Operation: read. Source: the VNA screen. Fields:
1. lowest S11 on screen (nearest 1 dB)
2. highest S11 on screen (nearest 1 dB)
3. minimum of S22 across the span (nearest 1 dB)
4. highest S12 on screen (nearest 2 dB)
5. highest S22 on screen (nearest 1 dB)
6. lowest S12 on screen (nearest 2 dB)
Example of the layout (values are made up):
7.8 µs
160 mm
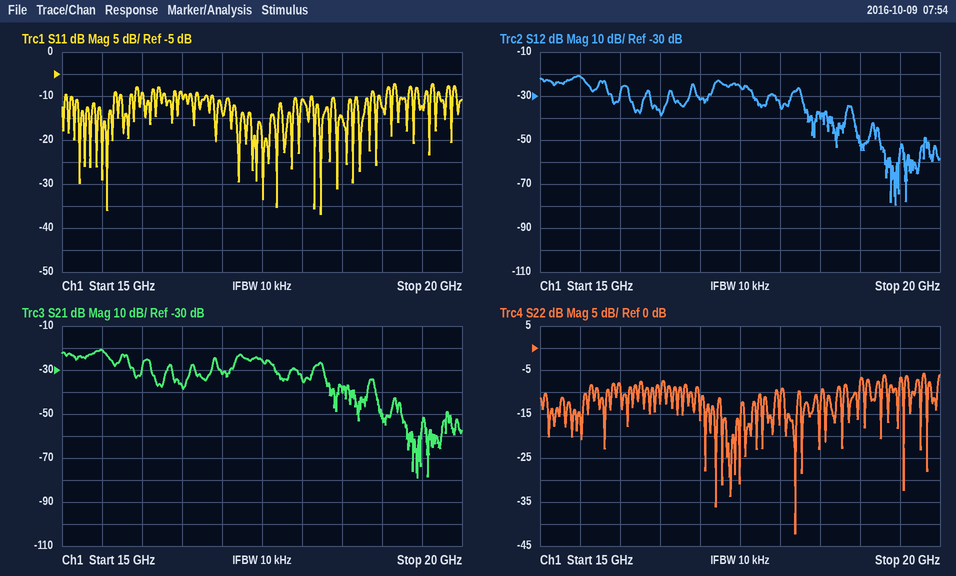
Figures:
-37 dB
-7 dB
-42 dB
-20 dB
-6 dB
-80 dB
